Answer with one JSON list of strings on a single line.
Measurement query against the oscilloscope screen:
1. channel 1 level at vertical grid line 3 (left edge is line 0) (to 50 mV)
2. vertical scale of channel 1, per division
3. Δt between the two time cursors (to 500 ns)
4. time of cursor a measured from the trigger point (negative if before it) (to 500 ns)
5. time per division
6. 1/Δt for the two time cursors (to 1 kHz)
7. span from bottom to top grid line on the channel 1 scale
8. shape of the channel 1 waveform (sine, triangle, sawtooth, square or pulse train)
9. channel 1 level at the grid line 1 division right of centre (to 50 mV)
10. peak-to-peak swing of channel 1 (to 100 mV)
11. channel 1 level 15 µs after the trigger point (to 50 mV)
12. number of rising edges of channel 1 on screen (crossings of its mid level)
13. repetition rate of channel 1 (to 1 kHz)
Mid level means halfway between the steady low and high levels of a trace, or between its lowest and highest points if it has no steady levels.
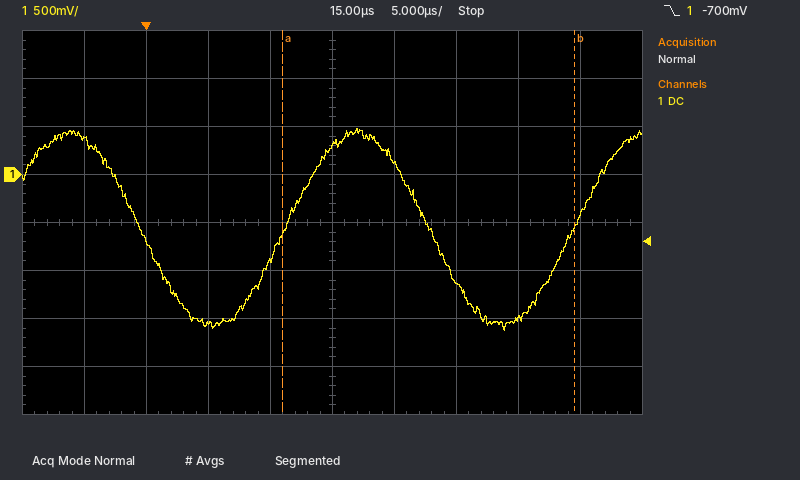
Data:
["-1.55 V", "500 mV", "23.5 µs", "+11.0 µs", "5 µs", "43 kHz", "4 V", "sine", "100 mV", "2.10 V", "300 mV", "2", "43 kHz"]
